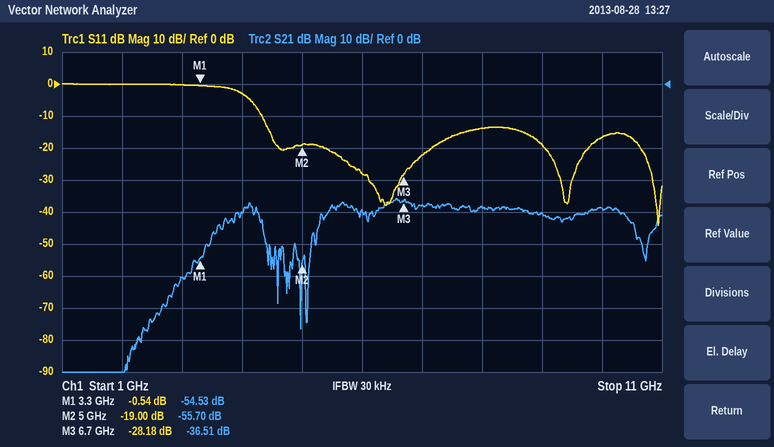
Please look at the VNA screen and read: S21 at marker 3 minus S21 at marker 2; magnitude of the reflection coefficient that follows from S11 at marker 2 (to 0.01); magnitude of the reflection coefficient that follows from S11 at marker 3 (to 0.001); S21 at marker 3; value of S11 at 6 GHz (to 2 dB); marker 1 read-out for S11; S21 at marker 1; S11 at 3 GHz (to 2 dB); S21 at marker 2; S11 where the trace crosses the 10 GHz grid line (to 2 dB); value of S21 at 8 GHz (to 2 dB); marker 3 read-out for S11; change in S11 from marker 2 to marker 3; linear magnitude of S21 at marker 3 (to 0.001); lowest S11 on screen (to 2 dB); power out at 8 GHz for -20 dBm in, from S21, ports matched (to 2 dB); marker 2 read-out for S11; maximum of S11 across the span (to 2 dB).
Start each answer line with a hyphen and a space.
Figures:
- 19.19 dB
- 0.11
- 0.039
- -36.51 dB
- -28 dB
- -0.54 dB
- -54.53 dB
- 0 dB
- -55.70 dB
- -16 dB
- -38 dB
- -28.18 dB
- -9.18 dB
- 0.015
- -44 dB
- -58 dBm
- -19.00 dB
- 0 dB
